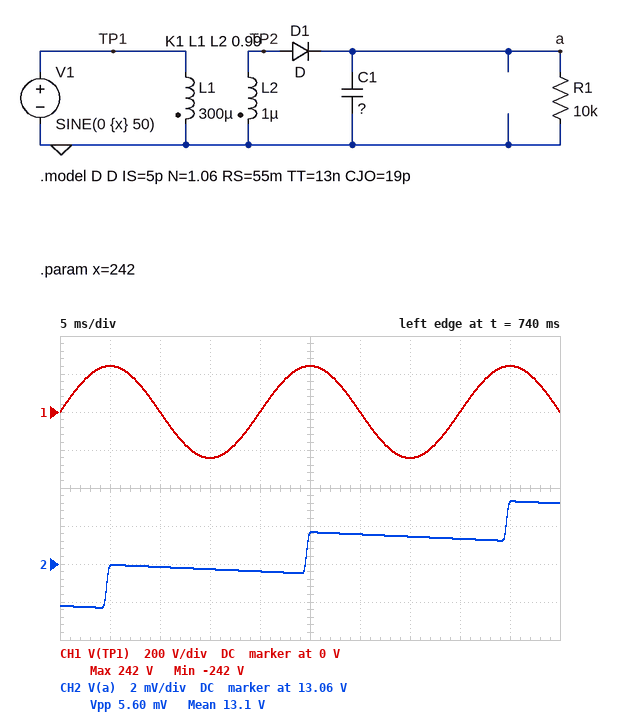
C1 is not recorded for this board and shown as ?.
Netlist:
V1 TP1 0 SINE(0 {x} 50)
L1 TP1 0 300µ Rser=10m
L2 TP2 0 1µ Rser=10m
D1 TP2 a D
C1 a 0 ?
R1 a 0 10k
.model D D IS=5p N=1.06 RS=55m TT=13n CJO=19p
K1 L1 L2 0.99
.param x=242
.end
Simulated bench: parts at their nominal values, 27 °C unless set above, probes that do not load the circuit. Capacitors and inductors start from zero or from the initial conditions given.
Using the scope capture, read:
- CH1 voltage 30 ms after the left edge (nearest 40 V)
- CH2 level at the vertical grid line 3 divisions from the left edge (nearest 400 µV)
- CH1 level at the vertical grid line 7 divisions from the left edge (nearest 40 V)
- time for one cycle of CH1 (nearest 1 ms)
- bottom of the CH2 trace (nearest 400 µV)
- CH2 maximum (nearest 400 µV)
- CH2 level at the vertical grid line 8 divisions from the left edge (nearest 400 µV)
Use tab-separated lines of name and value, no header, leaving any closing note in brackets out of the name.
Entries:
CH1 voltage 30 ms after the left edge	0 V
CH2 level at the vertical grid line 3 divisions from the left edge	13.0556 V
CH1 level at the vertical grid line 7 divisions from the left edge	-240 V
time for one cycle of CH1	20 ms
bottom of the CH2 trace	13.0536 V
CH2 maximum	13.0592 V
CH2 level at the vertical grid line 8 divisions from the left edge	13.0572 V
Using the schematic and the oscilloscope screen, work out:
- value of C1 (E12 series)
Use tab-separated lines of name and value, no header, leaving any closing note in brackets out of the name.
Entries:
value of C1	56 mF
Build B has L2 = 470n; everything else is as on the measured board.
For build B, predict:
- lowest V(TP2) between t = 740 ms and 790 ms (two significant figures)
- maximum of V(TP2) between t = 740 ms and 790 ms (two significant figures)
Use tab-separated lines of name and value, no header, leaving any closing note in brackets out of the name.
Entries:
lowest V(TP2) between t = 740 ms and 790 ms	-9.4 V
maximum of V(TP2) between t = 740 ms and 790 ms	9.4 V
